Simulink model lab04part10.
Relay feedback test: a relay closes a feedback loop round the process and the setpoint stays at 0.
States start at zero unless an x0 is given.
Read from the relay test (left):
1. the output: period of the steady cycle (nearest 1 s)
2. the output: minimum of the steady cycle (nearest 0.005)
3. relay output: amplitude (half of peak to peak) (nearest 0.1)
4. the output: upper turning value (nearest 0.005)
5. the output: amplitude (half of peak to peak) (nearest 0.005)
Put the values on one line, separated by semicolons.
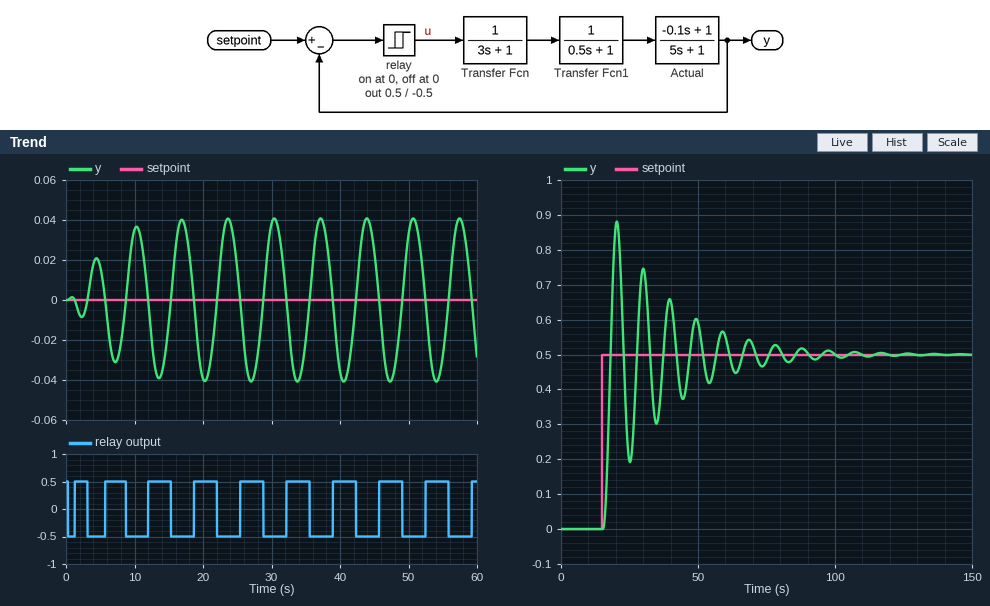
7 s; -0.040; 0.5; 0.040; 0.040
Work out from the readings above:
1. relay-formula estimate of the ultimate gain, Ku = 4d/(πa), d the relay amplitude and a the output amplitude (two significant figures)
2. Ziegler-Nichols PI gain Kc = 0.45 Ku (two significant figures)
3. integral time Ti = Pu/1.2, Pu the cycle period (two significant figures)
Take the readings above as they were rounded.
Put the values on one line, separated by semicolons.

16; 7.2; 5.8 s
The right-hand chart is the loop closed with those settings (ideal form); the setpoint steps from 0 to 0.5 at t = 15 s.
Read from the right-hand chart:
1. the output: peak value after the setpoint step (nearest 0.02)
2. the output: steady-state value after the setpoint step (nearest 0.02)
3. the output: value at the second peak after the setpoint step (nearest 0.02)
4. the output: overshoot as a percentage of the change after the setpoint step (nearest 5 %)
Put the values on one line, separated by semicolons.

0.88; 0.50; 0.74; 75 %
